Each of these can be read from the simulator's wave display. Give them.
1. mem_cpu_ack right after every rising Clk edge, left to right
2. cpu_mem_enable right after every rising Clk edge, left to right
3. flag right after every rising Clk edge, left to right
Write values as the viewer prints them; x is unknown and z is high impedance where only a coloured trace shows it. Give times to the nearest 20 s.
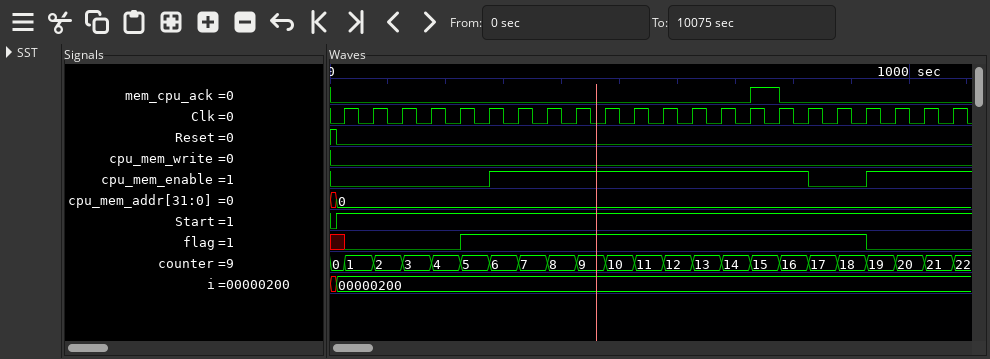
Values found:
0 0 0 0 0 0 0 0 0 0 0 0 0 0 1 0 0 0 0 0 0 0
0 0 0 0 0 1 1 1 1 1 1 1 1 1 1 1 0 0 1 1 1 1
0 0 0 0 1 1 1 1 1 1 1 1 1 1 1 1 1 1 0 0 0 0
